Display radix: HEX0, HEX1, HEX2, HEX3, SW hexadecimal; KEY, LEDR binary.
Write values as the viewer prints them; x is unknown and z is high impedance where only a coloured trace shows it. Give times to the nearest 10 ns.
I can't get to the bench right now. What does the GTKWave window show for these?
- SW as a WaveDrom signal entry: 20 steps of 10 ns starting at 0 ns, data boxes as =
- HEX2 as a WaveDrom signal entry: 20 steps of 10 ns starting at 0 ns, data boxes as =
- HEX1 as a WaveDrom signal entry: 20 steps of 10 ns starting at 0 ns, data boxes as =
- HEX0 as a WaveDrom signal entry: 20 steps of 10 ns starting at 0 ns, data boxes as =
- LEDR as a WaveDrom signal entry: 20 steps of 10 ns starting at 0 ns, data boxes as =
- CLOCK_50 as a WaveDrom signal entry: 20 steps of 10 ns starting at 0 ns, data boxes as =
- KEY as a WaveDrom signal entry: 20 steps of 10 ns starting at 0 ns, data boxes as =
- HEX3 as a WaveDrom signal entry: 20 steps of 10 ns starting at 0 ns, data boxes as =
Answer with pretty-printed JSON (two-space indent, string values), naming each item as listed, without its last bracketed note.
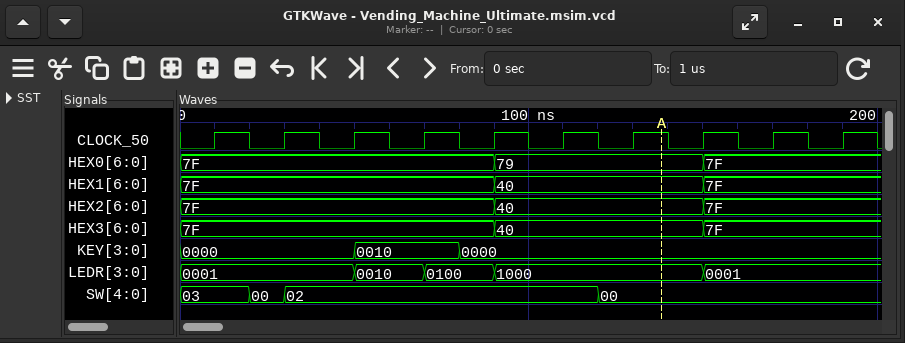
{
  "SW as a WaveDrom signal entry: 20 steps of 10 ns starting at 0 ns, data boxes as =": "{name: 'SW', wave: '=.==........=.......', data: '03 00 02 00'}",
  "HEX2 as a WaveDrom signal entry: 20 steps of 10 ns starting at 0 ns, data boxes as =": "{name: 'HEX2', wave: '=........=.....=....', data: '7F 40 7F'}",
  "HEX1 as a WaveDrom signal entry: 20 steps of 10 ns starting at 0 ns, data boxes as =": "{name: 'HEX1', wave: '=........=.....=....', data: '7F 40 7F'}",
  "HEX0 as a WaveDrom signal entry: 20 steps of 10 ns starting at 0 ns, data boxes as =": "{name: 'HEX0', wave: '=........=.....=....', data: '7F 79 7F'}",
  "LEDR as a WaveDrom signal entry: 20 steps of 10 ns starting at 0 ns, data boxes as =": "{name: 'LEDR', wave: '=....=.=.=.....=....', data: '0001 0010 0100 1000 0001'}",
  "CLOCK_50 as a WaveDrom signal entry: 20 steps of 10 ns starting at 0 ns, data boxes as =": "{name: 'CLOCK_50', wave: '01010101010101010101'}",
  "KEY as a WaveDrom signal entry: 20 steps of 10 ns starting at 0 ns, data boxes as =": "{name: 'KEY', wave: '=....=..=...........', data: '0000 0010 0000'}",
  "HEX3 as a WaveDrom signal entry: 20 steps of 10 ns starting at 0 ns, data boxes as =": "{name: 'HEX3', wave: '=........=.....=....', data: '7F 40 7F'}"
}
